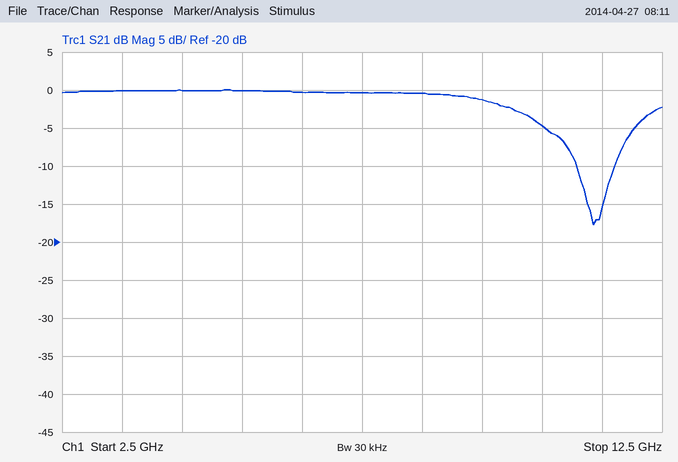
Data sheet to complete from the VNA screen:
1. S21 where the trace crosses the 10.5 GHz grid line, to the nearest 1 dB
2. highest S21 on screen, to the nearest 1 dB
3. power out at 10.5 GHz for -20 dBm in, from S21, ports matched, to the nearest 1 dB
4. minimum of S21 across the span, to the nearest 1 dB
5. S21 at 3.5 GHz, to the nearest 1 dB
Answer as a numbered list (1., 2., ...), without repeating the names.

1. -5 dB
2. 0 dB
3. -25 dBm
4. -18 dB
5. 0 dB
